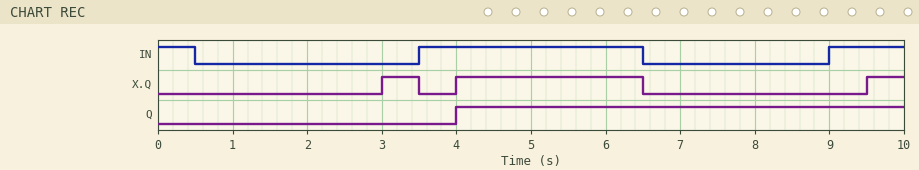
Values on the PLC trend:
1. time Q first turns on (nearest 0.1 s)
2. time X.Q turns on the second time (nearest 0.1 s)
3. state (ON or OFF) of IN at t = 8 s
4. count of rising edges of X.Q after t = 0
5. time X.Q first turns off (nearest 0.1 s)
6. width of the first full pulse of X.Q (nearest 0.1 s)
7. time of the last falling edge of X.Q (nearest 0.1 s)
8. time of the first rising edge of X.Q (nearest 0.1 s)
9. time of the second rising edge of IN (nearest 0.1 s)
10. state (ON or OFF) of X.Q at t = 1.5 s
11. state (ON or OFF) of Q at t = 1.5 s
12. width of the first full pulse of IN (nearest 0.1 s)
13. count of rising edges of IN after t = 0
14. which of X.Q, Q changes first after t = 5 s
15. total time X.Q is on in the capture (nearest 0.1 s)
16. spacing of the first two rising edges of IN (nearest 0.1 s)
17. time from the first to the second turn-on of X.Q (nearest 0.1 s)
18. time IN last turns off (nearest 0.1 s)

4.0 s
4.0 s
OFF
3
3.5 s
0.5 s
6.5 s
3.0 s
9.0 s
OFF
OFF
3.0 s
2
X.Q
3.5 s
5.5 s
1.0 s
6.5 s
